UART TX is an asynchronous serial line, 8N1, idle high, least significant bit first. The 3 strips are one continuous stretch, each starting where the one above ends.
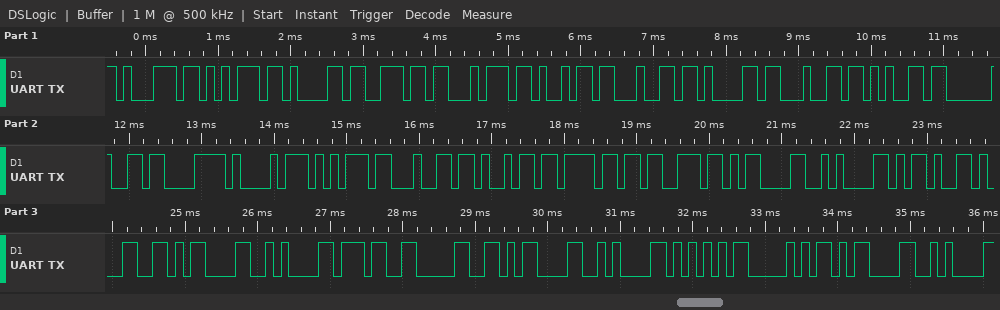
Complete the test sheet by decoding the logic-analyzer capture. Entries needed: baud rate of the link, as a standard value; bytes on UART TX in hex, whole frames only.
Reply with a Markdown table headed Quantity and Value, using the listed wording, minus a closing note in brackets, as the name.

| Quantity | Value |
|---|---|
| baud rate of the link, as a standard value | 9600 baud |
| bytes on UART TX in hex, whole frames only | 71 75 61 6E 74 69 64 61 64 65 20 C3 A1 75 64 69 6F 73 0D 0A 2D 31 0D 0A 37 30 0D 0A 55 50 0D 0A |
